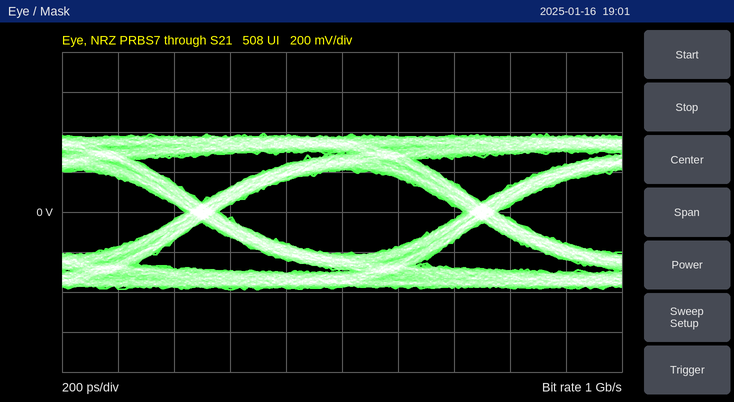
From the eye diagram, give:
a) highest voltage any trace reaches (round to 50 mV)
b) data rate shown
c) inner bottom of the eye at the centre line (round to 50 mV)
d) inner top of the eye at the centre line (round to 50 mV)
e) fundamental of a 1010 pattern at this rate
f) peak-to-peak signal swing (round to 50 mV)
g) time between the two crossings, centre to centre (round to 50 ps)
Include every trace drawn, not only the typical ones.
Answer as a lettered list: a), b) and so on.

a) 400 mV
b) 1 Gb/s
c) -200 mV
d) 200 mV
e) 500 MHz
f) 800 mV
g) 1.00 ns
